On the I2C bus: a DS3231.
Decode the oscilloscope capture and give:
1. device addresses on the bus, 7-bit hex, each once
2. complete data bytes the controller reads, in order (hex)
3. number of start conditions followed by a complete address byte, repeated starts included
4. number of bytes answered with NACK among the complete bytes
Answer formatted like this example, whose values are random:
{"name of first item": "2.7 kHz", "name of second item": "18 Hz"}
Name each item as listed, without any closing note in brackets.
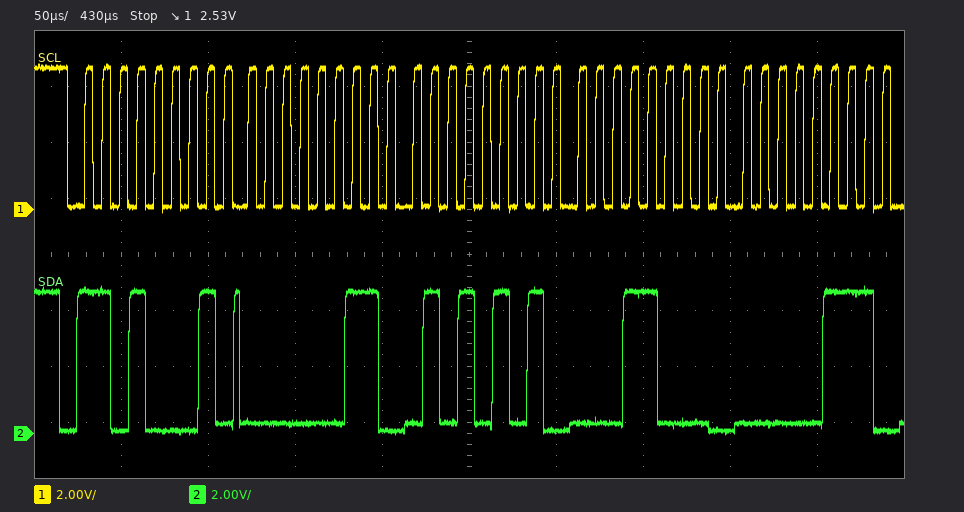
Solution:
{"device addresses on the bus, 7-bit hex, each once": "0x68", "complete data bytes the controller reads, in order": "03 55 18 07", "number of start conditions followed by a complete address byte, repeated starts included": "1", "number of bytes answered with NACK among the complete bytes": "0"}
